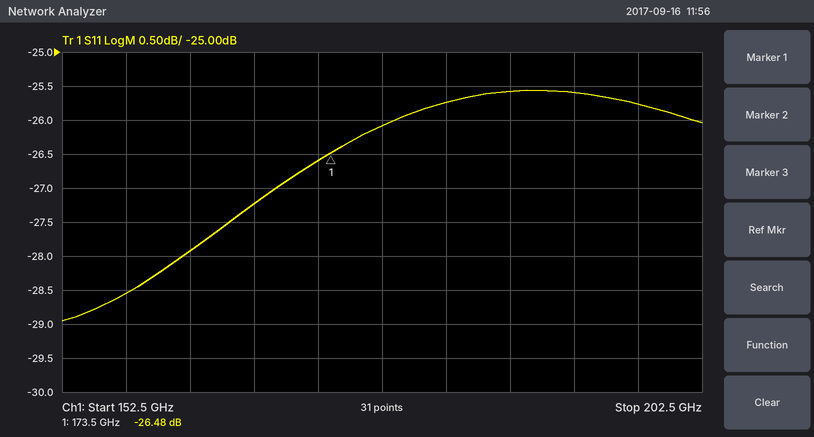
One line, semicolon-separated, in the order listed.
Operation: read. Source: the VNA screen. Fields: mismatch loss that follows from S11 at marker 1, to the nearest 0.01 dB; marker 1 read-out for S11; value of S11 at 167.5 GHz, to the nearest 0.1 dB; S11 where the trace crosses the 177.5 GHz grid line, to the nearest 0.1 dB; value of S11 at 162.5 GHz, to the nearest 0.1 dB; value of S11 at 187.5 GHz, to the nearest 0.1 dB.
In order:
0.01 dB; -26.48 dB; -27.2 dB; -26.1 dB; -27.9 dB; -25.6 dB
